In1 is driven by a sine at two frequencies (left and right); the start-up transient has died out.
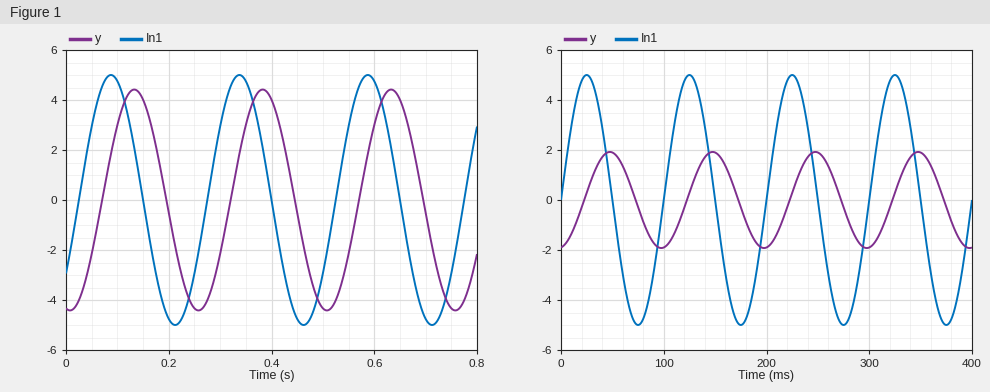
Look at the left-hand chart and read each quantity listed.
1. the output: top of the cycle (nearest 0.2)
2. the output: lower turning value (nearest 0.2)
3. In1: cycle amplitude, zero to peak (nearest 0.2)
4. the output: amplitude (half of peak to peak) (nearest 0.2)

4.4
-4.4
5.0
4.4
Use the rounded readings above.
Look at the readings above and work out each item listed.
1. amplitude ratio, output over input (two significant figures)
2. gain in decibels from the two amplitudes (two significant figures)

0.88
-1.1 dB
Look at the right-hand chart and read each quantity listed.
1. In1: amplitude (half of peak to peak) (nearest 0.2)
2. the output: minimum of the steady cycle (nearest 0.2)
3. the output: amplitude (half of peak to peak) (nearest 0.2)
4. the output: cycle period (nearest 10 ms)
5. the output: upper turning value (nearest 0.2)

5.0
-2.0
2.0
100 ms
2.0
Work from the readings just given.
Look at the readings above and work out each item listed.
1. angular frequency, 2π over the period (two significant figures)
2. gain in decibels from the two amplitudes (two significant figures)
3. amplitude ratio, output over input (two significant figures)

0.063 rad/ms
-8.0 dB
0.40
